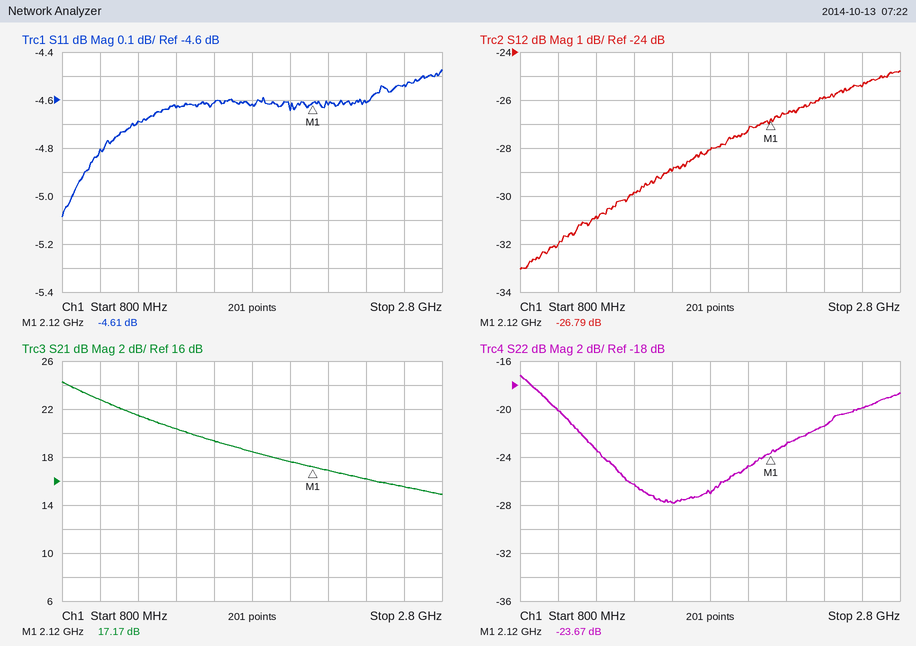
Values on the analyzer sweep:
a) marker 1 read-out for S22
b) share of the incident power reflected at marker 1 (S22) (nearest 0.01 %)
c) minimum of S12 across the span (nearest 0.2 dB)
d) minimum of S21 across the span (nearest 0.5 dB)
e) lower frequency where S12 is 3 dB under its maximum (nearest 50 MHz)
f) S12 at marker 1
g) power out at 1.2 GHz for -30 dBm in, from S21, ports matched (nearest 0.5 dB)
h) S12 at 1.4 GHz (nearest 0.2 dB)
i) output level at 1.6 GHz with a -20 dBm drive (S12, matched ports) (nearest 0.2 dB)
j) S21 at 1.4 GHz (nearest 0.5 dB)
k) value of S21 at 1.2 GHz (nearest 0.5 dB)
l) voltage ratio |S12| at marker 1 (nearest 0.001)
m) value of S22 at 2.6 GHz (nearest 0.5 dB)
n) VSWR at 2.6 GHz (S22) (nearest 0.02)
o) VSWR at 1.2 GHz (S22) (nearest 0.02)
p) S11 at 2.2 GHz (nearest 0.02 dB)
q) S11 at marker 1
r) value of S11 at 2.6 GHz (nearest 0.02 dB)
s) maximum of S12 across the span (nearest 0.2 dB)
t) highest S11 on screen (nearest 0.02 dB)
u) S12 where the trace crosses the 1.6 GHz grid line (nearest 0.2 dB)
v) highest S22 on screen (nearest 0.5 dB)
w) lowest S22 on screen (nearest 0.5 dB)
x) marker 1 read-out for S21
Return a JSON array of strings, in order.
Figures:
["-23.67 dB", "0.43 %", "-33.0 dB", "15.0 dB", "1.90 GHz", "-26.79 dB", "-8.5 dBm", "-29.8 dB", "-49.0 dBm", "20.5 dB", "21.5 dB", "0.046", "-20.0 dB", "1.22", "1.14", "-4.62 dB", "-4.61 dB", "-4.54 dB", "-24.8 dB", "-4.48 dB", "-29.0 dB", "-17.0 dB", "-28.0 dB", "17.17 dB"]
